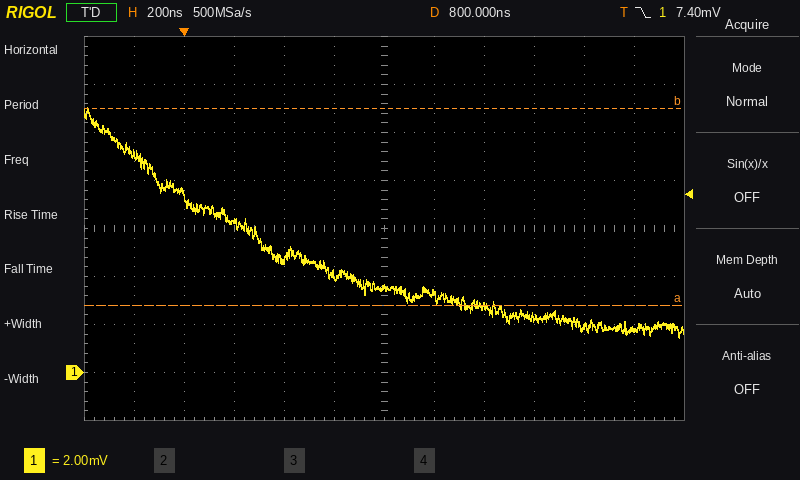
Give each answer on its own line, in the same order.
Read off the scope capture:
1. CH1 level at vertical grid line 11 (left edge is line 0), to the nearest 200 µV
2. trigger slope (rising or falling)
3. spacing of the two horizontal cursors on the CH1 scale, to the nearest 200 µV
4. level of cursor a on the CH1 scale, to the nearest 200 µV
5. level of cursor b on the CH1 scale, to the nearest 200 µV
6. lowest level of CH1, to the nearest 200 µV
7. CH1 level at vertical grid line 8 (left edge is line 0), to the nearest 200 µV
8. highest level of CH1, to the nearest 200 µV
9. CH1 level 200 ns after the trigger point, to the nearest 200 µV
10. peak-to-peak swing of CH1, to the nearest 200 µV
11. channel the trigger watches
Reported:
1.8 mV
falling
8.2 mV
2.8 mV
11.0 mV
1.4 mV
2.8 mV
11.0 mV
6.2 mV
9.6 mV
CH1
